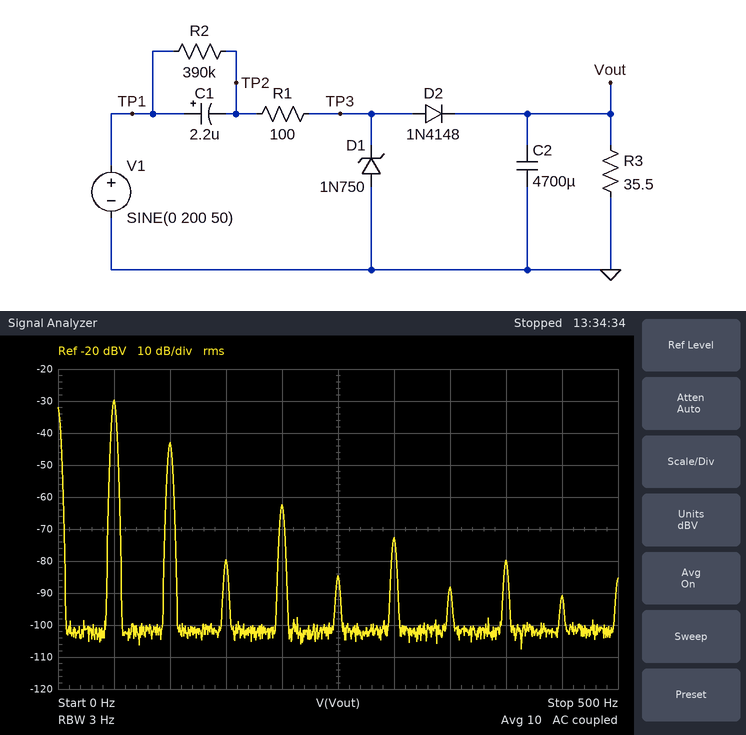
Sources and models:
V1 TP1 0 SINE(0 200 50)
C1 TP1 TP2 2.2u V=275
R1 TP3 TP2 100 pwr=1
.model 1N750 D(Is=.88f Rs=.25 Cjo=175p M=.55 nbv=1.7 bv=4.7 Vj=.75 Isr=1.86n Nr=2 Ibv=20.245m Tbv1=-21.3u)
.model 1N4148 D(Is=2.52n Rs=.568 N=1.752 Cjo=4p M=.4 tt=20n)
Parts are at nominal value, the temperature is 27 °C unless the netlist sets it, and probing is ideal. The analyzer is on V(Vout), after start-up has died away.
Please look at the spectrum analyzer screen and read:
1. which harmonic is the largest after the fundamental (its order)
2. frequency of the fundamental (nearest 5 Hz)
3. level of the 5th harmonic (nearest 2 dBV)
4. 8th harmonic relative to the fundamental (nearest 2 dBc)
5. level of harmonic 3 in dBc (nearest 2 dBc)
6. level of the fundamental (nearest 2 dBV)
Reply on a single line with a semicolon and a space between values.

2; 50 Hz; -84 dBV; -50 dBc; -50 dBc; -30 dBV
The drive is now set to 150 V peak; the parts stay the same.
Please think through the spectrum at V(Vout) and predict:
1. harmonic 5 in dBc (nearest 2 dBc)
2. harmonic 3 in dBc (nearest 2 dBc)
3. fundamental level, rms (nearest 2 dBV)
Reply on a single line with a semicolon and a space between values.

-54 dBc; -48 dBc; -32 dBV
